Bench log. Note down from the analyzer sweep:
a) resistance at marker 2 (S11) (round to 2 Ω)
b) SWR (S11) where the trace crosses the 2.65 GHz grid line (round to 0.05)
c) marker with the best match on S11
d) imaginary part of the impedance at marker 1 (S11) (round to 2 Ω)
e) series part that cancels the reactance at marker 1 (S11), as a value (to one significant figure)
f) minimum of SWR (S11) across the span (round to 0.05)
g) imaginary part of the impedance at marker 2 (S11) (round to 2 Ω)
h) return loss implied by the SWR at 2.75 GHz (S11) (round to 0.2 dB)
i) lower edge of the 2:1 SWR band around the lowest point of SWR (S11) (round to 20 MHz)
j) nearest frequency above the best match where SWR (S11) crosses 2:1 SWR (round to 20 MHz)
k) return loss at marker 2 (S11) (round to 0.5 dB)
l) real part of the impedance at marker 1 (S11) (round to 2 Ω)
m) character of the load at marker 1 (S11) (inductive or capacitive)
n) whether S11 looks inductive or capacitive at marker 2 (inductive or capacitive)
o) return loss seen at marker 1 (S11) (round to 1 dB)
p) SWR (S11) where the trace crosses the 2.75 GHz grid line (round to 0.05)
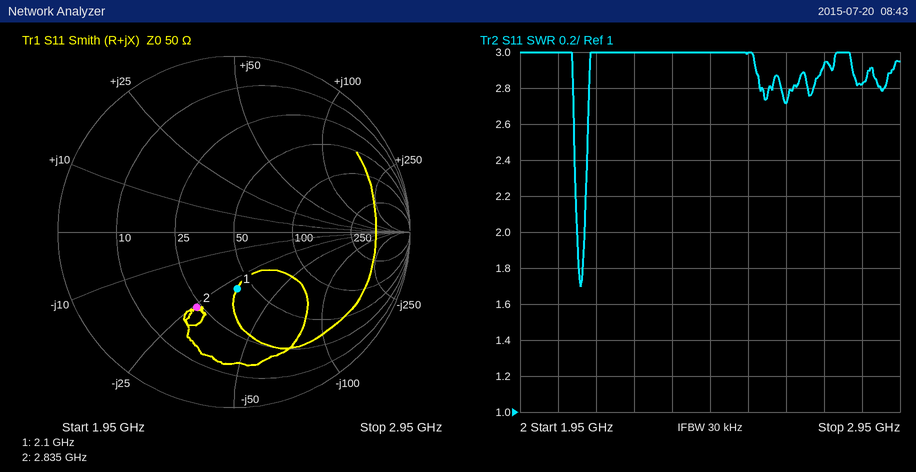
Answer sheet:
24 Ω
2.70
marker 1
-30 Ω
2 nH
1.70
-26 Ω
6.2 dB
2.10 GHz
2.12 GHz
6.5 dB
42 Ω
capacitive
capacitive
10 dB
2.95
